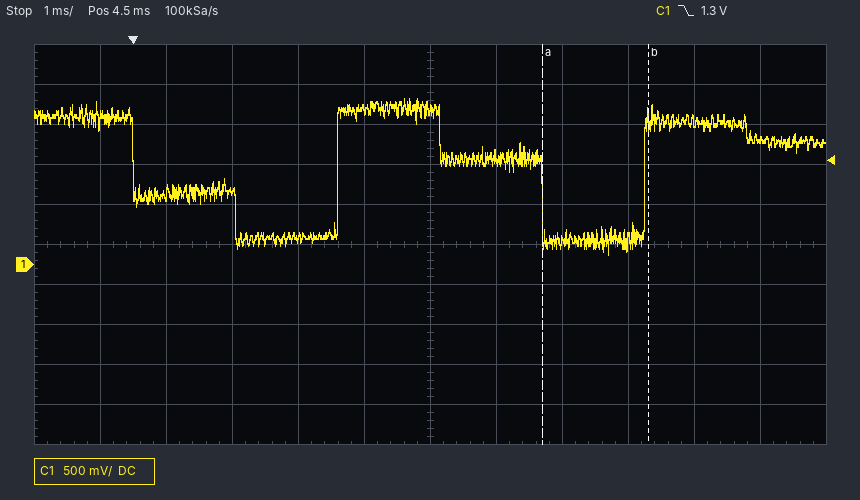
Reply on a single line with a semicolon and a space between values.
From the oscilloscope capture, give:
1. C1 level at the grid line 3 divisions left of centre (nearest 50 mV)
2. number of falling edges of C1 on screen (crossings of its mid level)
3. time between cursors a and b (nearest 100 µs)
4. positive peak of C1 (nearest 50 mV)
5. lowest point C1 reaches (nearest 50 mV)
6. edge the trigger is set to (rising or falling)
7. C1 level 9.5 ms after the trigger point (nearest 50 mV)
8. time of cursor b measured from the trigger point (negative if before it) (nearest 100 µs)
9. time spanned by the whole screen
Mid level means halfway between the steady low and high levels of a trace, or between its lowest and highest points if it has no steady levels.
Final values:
900 mV; 2; 1.6 ms; 2.10 V; 100 mV; falling; 1.55 V; +7.8 ms; 12 ms
